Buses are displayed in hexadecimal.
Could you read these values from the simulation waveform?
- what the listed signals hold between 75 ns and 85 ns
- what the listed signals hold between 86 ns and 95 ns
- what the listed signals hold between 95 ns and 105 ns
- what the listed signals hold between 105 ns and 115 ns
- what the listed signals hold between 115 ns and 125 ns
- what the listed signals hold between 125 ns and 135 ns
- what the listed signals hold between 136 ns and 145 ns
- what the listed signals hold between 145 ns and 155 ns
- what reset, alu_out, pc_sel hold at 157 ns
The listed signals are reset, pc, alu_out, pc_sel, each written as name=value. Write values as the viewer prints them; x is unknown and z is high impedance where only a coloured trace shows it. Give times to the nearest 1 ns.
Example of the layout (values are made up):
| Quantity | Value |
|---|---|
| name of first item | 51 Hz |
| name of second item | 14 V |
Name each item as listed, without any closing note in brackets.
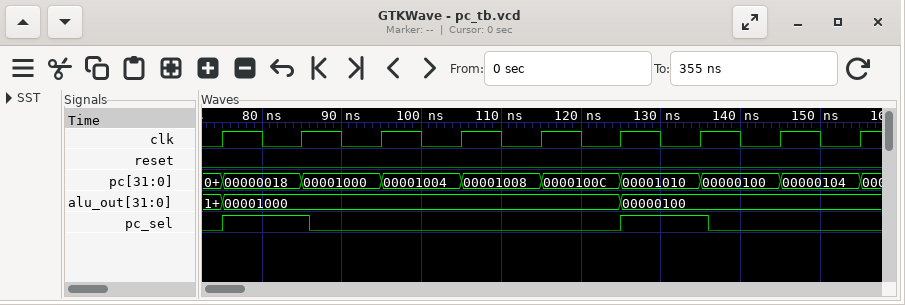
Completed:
| Quantity | Value |
|---|---|
| what the listed signals hold between 75 ns and 85 ns | reset=0, pc=00000018, alu_out=00001000, pc_sel=1 |
| what the listed signals hold between 86 ns and 95 ns | reset=0, pc=00001000, alu_out=00001000, pc_sel=0 |
| what the listed signals hold between 95 ns and 105 ns | reset=0, pc=00001004, alu_out=00001000, pc_sel=0 |
| what the listed signals hold between 105 ns and 115 ns | reset=0, pc=00001008, alu_out=00001000, pc_sel=0 |
| what the listed signals hold between 115 ns and 125 ns | reset=0, pc=0000100C, alu_out=00001000, pc_sel=0 |
| what the listed signals hold between 125 ns and 135 ns | reset=0, pc=00001010, alu_out=00000100, pc_sel=1 |
| what the listed signals hold between 136 ns and 145 ns | reset=0, pc=00000100, alu_out=00000100, pc_sel=0 |
| what the listed signals hold between 145 ns and 155 ns | reset=0, pc=00000104, alu_out=00000100, pc_sel=0 |
| what reset, alu_out, pc_sel hold at 157 ns | reset=0, alu_out=00000100, pc_sel=0 |
